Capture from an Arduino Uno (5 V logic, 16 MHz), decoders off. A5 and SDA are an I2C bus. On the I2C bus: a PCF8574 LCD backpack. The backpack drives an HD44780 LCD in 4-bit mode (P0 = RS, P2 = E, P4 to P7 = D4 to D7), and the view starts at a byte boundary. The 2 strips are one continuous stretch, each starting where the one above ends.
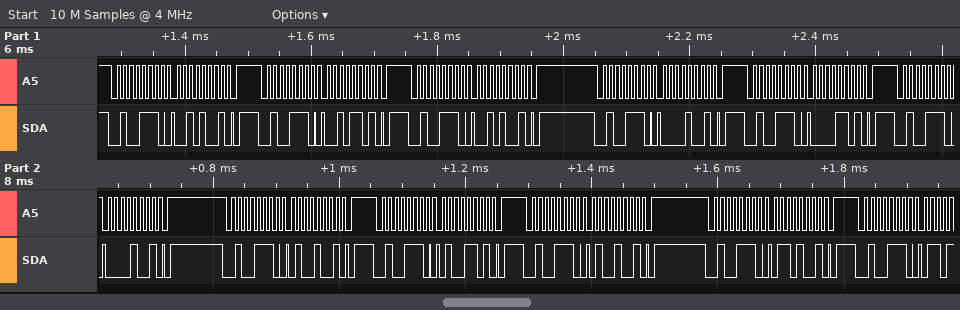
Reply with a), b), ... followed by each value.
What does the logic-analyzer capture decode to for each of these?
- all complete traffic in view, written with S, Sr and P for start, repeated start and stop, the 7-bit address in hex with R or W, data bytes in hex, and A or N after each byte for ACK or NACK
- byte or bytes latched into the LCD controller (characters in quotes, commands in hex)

a) S 27W A 29 A P S 27W A 2D A P S 27W A 29 A P S 27W A 09 A P S 27W A 0D A P S 27W A 09 A P S 27W A 49 A P S 27W A 4D A P S 27W A 49 A P S 27W A 69 A P S 27W A
b) ' '
